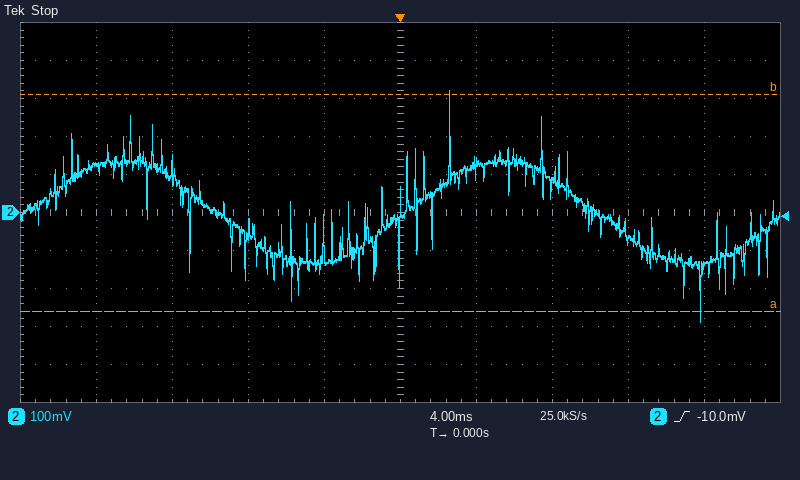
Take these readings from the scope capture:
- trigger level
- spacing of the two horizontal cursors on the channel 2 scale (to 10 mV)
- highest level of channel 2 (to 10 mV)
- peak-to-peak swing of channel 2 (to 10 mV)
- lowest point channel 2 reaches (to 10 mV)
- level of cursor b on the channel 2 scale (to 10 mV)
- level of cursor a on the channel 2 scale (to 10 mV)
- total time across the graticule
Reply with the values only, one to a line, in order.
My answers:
-10.0 mV
570 mV
320 mV
610 mV
-290 mV
310 mV
-260 mV
40 ms
